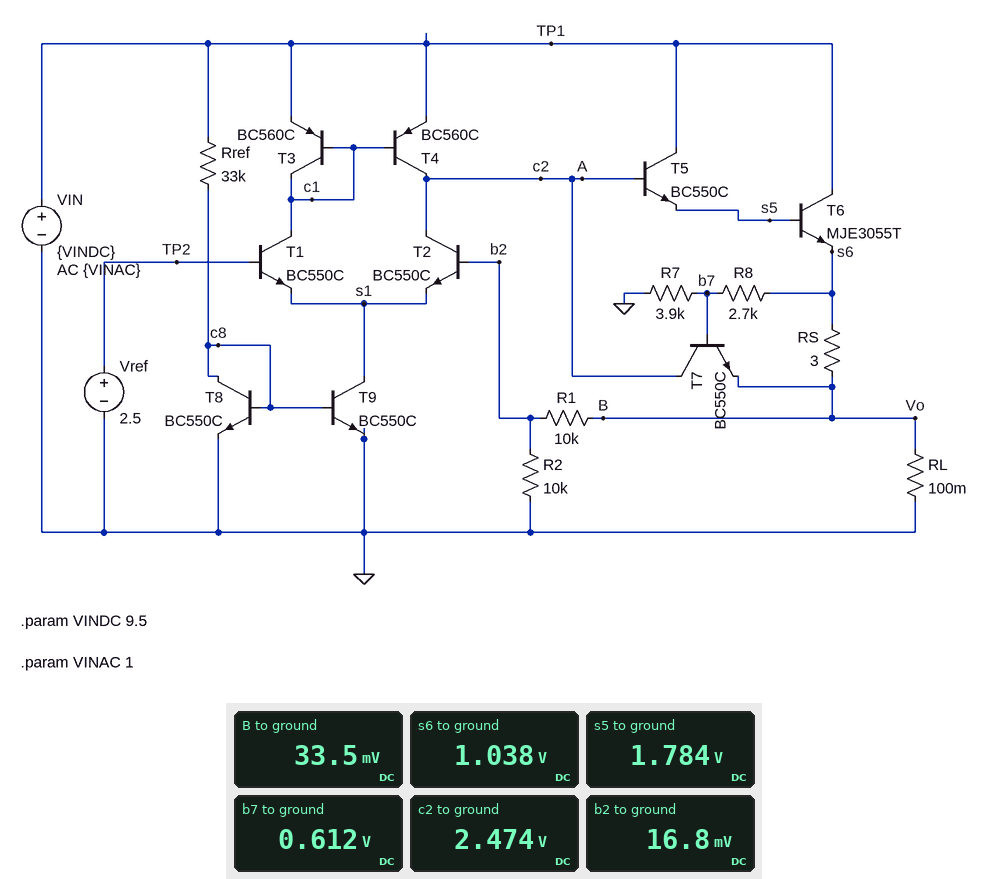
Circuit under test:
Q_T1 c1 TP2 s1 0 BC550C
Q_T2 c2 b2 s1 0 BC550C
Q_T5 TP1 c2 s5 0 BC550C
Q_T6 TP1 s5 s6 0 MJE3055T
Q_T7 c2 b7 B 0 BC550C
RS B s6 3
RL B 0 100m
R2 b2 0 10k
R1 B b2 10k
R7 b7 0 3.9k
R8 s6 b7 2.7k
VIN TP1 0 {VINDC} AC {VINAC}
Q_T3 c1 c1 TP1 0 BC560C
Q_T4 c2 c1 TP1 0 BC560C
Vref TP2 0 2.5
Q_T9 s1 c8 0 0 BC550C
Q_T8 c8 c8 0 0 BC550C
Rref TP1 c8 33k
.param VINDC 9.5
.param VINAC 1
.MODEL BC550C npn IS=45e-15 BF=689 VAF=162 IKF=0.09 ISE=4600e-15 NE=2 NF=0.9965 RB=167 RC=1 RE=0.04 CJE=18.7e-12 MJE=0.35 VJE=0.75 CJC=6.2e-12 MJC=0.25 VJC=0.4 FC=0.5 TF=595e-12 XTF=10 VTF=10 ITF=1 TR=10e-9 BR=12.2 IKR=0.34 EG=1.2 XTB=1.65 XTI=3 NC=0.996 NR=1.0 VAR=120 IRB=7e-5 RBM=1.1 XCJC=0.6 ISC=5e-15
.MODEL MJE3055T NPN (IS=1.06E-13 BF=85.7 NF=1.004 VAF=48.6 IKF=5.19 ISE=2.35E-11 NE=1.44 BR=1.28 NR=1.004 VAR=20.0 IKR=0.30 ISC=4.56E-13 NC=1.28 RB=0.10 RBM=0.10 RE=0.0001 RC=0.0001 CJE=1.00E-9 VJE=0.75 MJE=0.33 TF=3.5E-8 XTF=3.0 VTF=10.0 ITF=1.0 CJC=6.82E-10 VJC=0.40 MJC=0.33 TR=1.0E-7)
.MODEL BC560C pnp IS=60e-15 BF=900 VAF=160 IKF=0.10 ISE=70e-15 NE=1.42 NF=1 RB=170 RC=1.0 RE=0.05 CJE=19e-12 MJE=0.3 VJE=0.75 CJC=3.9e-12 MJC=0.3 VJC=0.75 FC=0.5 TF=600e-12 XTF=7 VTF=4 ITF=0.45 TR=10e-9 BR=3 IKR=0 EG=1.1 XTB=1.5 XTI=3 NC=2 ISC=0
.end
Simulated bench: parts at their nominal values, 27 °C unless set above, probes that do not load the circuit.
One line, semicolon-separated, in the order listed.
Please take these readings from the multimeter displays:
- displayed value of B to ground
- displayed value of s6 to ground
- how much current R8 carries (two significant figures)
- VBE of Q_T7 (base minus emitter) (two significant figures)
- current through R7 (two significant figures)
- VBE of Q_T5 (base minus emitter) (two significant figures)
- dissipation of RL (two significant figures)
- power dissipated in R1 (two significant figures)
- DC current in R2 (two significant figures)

33.5 mV; 1.038 V; 160 µA; 580 mV; 160 µA; 690 mV; 11 mW; 28 nW; 1.7 µA
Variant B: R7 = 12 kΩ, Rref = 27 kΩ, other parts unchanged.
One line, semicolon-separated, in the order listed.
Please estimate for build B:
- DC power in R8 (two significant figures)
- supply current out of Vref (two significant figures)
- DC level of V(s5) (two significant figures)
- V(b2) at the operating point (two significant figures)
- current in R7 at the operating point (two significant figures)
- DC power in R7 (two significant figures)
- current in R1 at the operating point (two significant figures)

7.2 µW; 840 nA; 1.5 V; 12 mV; 51 µA; 31 µW; 1.2 µA
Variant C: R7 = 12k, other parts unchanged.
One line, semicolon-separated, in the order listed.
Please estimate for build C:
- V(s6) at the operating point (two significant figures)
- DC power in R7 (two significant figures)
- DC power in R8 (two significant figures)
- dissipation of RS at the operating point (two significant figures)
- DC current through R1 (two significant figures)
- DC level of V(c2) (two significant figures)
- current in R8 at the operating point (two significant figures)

740 mV; 30 µW; 7.0 µW; 170 mW; 1.2 µA; 2.2 V; 51 µA
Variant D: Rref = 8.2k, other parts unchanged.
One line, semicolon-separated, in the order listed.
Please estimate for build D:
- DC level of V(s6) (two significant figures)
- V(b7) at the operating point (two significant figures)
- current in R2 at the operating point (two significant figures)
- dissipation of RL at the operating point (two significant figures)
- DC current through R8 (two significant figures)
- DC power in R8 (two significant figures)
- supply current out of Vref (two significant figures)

1.1 V; 650 mV; 1.8 µA; 13 mW; 170 µA; 78 µW; 2.2 µA
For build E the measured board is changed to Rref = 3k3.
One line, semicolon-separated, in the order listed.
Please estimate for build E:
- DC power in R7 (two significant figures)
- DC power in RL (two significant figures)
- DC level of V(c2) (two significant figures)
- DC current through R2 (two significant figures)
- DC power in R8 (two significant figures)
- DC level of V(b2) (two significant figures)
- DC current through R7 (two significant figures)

120 µW; 14 mW; 2.6 V; 1.9 µA; 87 µW; 19 mV; 170 µA
